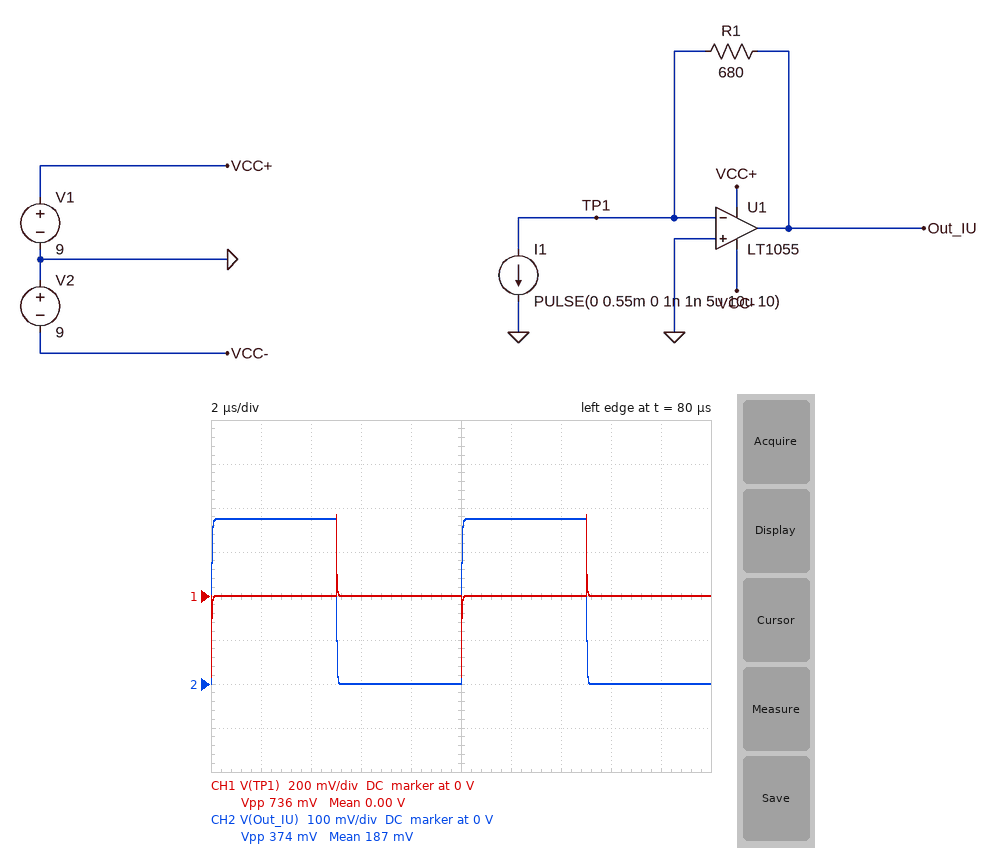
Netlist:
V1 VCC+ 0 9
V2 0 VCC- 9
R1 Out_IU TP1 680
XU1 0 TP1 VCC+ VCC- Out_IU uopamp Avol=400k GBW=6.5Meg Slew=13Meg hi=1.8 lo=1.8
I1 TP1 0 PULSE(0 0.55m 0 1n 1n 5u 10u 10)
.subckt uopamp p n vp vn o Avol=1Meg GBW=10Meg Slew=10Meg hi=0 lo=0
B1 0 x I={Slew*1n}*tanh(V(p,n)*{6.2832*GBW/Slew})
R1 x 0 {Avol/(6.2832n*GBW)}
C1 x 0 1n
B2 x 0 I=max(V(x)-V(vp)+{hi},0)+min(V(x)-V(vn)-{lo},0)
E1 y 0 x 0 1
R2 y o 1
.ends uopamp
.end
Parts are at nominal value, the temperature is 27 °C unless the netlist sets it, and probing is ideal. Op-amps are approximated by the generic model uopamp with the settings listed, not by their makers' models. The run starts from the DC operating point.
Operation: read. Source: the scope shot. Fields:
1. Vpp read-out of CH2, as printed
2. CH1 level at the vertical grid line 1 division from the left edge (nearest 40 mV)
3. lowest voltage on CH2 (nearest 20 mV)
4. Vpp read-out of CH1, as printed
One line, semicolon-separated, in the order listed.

374 mV; 0 V; 0 V; 736 mV
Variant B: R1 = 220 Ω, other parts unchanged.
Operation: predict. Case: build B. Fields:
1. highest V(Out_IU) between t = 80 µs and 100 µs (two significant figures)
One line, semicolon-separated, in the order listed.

120 mV
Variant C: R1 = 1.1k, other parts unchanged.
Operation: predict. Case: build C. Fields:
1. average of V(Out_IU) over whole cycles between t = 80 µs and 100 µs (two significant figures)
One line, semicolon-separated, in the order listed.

300 mV
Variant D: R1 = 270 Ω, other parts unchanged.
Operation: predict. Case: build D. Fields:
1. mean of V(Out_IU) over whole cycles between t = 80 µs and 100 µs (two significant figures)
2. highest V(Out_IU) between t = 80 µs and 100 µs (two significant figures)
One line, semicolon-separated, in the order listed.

74 mV; 150 mV
